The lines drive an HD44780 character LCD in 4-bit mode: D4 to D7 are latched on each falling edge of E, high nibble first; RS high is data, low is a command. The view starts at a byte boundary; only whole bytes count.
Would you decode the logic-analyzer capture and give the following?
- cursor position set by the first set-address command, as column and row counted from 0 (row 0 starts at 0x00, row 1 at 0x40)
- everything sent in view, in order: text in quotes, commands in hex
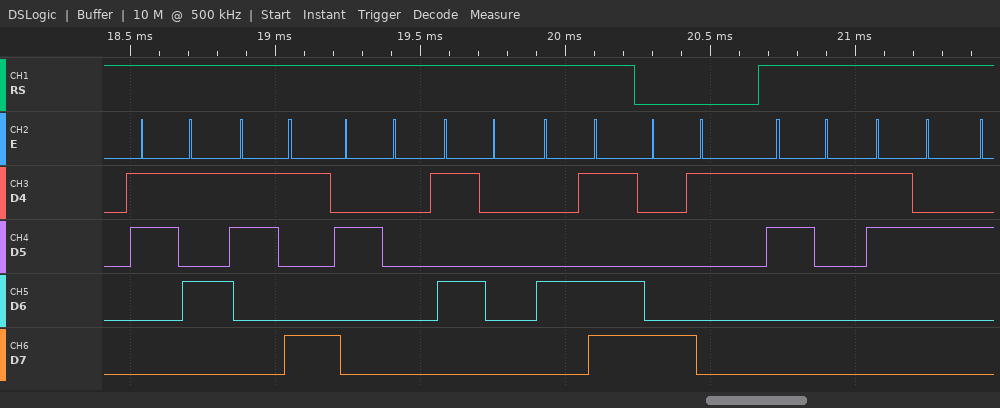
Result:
column 1, row 0
"59 PM" 0x81 "12"
